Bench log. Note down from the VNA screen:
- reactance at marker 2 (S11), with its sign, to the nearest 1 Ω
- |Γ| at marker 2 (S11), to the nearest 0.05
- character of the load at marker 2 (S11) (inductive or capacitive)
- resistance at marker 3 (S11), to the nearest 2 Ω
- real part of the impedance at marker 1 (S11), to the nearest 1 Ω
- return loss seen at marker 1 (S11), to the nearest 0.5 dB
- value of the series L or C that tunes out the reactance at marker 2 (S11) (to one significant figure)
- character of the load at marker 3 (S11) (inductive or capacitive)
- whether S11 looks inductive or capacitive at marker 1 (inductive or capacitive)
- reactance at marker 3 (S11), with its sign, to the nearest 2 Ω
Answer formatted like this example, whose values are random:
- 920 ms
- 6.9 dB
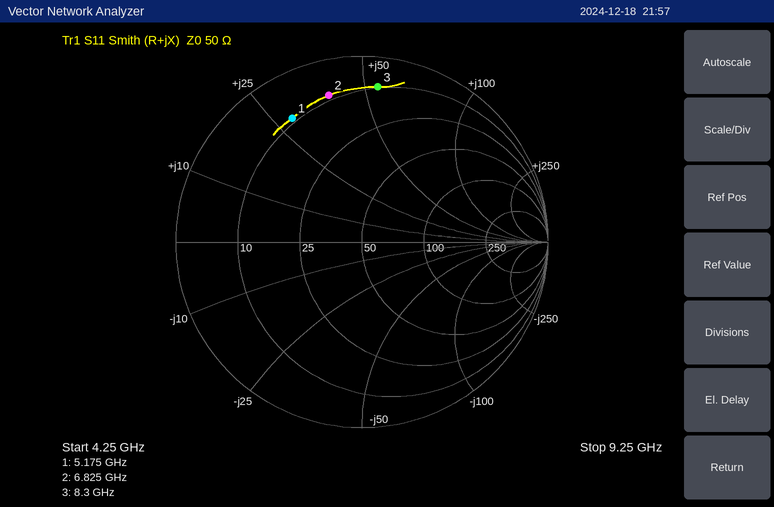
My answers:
- +39 Ω
- 0.80
- inductive
- 10 Ω
- 9 Ω
- 2.5 dB
- 600 fF
- inductive
- inductive
- +54 Ω
